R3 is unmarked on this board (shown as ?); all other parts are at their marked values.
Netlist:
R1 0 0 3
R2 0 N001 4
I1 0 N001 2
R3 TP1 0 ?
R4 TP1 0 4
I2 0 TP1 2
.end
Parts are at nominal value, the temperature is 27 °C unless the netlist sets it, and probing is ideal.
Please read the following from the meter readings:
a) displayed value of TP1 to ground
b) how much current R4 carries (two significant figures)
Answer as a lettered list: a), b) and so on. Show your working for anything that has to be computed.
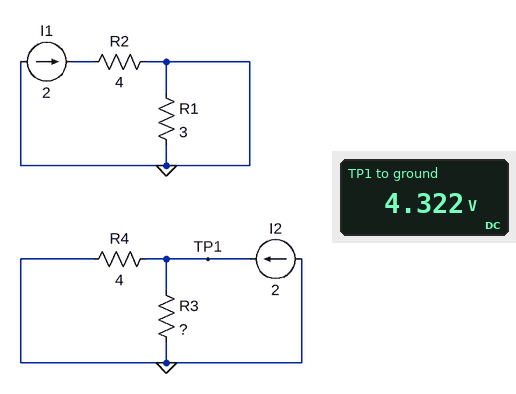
a) 4.322 V
b) (4.322 V) / 4 Ω = 1.1 A
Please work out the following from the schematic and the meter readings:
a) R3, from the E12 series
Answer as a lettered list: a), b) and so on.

a) 4.7 Ω
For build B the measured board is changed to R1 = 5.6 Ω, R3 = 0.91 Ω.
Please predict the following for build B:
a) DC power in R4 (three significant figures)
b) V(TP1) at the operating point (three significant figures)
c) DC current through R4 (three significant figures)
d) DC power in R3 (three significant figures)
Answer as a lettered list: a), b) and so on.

a) 550 mW
b) 1.48 V
c) 371 mA
d) 2.42 W
